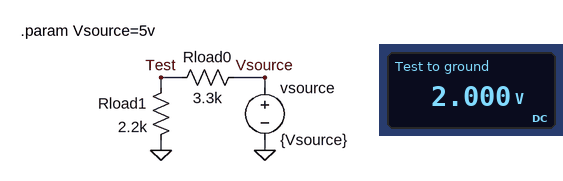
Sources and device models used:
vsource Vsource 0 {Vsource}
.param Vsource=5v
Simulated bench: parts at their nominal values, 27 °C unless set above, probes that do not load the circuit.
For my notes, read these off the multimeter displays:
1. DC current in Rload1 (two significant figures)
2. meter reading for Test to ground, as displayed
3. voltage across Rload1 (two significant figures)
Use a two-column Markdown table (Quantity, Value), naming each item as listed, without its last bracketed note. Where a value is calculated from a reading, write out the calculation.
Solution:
| Quantity | Value |
|---|---|
| DC current in Rload1 | (2 V) / 2.2 kΩ = 910 µA |
| meter reading for Test to ground, as displayed | 2.000 V |
| voltage across Rload1 | 2 V = 2.0 V |
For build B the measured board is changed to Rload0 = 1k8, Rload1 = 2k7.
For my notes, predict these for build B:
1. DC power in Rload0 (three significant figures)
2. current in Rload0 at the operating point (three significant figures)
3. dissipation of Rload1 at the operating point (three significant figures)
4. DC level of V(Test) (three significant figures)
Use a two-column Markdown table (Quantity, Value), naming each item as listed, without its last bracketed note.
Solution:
| Quantity | Value |
|---|---|
| DC power in Rload0 | 2.22 mW |
| current in Rload0 at the operating point | 1.11 mA |
| dissipation of Rload1 at the operating point | 3.33 mW |
| DC level of V(Test) | 3.00 V |
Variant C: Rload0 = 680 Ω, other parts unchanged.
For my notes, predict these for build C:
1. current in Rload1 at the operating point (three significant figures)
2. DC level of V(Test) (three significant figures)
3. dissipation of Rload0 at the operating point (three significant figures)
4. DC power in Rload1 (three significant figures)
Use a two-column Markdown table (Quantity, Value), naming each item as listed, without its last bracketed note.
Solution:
| Quantity | Value |
|---|---|
| current in Rload1 at the operating point | 1.74 mA |
| DC level of V(Test) | 3.82 V |
| dissipation of Rload0 at the operating point | 2.05 mW |
| DC power in Rload1 | 6.63 mW |
